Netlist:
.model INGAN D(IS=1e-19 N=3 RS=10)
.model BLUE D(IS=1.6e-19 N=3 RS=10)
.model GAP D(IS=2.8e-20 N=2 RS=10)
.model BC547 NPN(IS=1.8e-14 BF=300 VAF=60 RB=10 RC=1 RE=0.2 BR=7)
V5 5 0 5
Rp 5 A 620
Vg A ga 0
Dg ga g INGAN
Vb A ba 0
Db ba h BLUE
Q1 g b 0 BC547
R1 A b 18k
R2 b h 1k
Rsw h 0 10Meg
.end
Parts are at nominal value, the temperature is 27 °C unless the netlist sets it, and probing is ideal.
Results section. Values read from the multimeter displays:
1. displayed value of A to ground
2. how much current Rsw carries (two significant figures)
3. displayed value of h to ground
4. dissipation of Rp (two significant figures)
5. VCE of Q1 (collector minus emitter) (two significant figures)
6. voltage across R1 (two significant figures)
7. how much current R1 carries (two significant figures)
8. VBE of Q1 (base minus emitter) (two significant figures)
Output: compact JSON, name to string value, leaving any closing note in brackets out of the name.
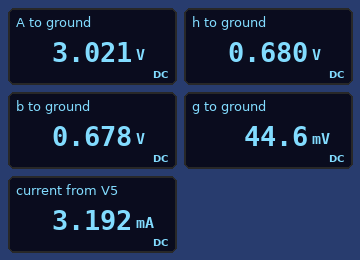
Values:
{"displayed value of A to ground": "3.021 V", "how much current Rsw carries": "68 nA", "displayed value of h to ground": "0.680 V", "dissipation of Rp": "6.3 mW", "VCE of Q1 (collector minus emitter)": "45 mV", "voltage across R1": "2.3 V", "how much current R1 carries": "130 µA", "VBE of Q1 (base minus emitter)": "680 mV"}
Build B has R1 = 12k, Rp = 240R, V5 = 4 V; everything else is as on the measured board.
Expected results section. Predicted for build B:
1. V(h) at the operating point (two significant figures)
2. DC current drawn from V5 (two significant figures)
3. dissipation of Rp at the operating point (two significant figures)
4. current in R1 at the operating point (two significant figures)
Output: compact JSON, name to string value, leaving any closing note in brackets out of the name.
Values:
{"V(h) at the operating point": "690 mV", "DC current drawn from V5": "4.0 mA", "dissipation of Rp at the operating point": "3.8 mW", "current in R1 at the operating point": "200 µA"}
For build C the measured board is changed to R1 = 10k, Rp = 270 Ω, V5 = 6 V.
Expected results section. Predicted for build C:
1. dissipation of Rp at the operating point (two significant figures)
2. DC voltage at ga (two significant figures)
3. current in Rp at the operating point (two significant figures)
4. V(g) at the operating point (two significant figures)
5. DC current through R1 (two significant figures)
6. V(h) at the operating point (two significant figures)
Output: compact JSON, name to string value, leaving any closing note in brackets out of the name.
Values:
{"dissipation of Rp at the operating point": "29 mW", "DC voltage at ga": "3.2 V", "current in Rp at the operating point": "10 mA", "V(g) at the operating point": "65 mV", "DC current through R1": "250 µA", "V(h) at the operating point": "720 mV"}
